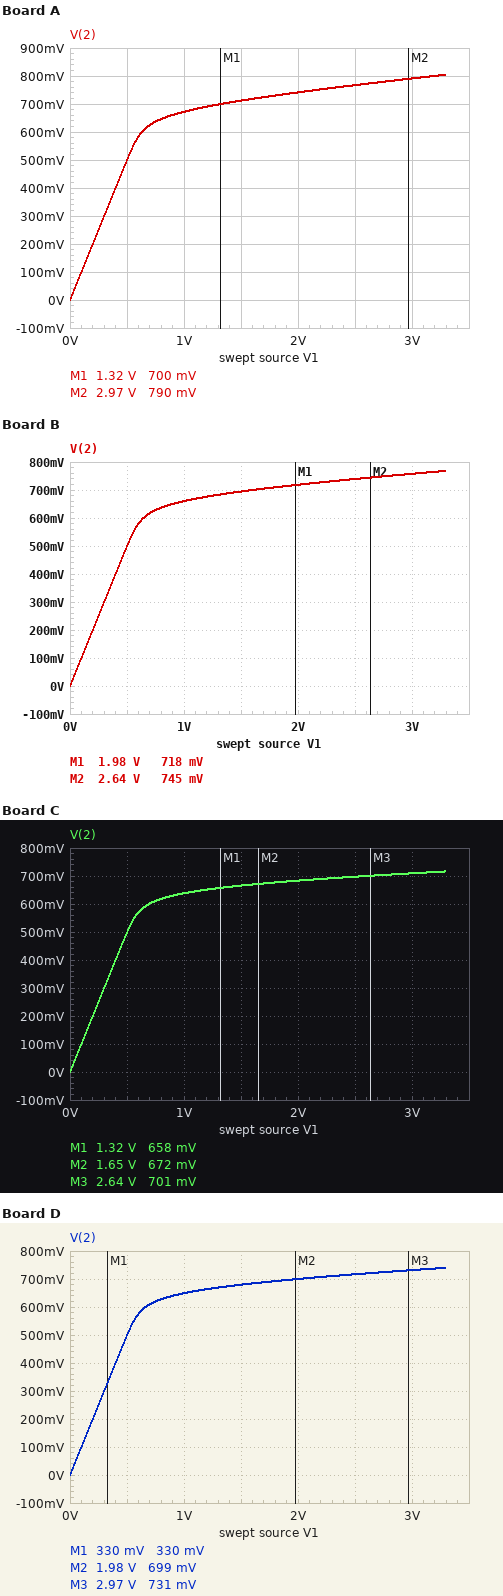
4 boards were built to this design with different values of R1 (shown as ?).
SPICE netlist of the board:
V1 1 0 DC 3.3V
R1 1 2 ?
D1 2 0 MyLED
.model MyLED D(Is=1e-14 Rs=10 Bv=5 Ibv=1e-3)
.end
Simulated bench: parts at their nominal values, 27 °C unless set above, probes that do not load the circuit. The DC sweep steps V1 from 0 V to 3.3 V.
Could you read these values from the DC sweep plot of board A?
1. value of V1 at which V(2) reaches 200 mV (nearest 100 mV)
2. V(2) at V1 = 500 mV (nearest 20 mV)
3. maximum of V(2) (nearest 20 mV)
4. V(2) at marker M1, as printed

200 mV
500 mV
800 mV
700 mV
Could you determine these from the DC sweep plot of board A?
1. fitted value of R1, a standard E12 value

270 Ω
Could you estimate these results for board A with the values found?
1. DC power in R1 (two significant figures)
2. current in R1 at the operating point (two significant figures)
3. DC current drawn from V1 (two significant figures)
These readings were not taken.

23 mW
9.2 mA
9.2 mA
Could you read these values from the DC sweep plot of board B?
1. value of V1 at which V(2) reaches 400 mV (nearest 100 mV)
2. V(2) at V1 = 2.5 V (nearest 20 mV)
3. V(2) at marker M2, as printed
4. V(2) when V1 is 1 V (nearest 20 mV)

400 mV
740 mV
745 mV
660 mV
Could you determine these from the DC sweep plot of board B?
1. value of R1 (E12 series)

390 Ω
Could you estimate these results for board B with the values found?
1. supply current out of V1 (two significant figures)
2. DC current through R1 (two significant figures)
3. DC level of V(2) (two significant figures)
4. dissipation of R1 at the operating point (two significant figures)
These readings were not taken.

6.5 mA
6.5 mA
770 mV
16 mW
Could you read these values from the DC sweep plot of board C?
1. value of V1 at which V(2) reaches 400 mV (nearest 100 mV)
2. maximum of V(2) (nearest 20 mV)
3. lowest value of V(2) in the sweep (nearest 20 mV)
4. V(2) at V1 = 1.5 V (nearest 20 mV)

400 mV
720 mV
0 V
660 mV
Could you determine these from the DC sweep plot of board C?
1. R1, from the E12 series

820 Ω
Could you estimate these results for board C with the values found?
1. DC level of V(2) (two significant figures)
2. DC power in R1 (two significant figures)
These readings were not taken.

720 mV
8.1 mW
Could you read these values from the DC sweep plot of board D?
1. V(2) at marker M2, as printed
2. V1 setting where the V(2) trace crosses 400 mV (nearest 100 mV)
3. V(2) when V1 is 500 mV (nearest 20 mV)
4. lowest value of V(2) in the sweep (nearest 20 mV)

699 mV
400 mV
500 mV
0 V
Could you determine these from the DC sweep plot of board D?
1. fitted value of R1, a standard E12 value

560 Ω
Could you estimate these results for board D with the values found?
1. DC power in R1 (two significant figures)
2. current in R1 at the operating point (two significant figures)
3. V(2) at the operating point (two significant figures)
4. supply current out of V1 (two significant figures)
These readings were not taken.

12 mW
4.6 mA
740 mV
4.6 mA
